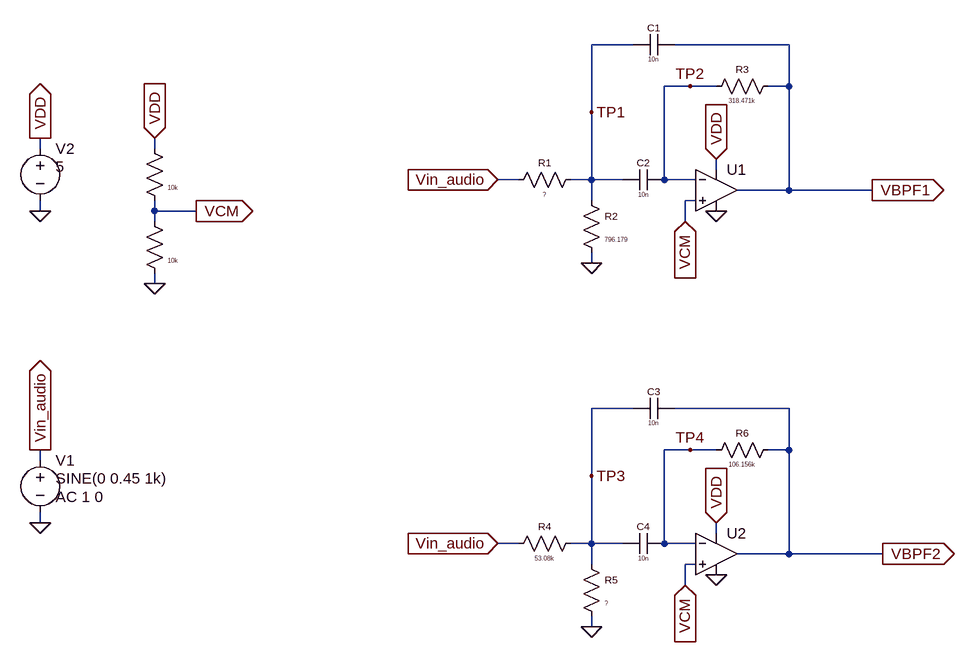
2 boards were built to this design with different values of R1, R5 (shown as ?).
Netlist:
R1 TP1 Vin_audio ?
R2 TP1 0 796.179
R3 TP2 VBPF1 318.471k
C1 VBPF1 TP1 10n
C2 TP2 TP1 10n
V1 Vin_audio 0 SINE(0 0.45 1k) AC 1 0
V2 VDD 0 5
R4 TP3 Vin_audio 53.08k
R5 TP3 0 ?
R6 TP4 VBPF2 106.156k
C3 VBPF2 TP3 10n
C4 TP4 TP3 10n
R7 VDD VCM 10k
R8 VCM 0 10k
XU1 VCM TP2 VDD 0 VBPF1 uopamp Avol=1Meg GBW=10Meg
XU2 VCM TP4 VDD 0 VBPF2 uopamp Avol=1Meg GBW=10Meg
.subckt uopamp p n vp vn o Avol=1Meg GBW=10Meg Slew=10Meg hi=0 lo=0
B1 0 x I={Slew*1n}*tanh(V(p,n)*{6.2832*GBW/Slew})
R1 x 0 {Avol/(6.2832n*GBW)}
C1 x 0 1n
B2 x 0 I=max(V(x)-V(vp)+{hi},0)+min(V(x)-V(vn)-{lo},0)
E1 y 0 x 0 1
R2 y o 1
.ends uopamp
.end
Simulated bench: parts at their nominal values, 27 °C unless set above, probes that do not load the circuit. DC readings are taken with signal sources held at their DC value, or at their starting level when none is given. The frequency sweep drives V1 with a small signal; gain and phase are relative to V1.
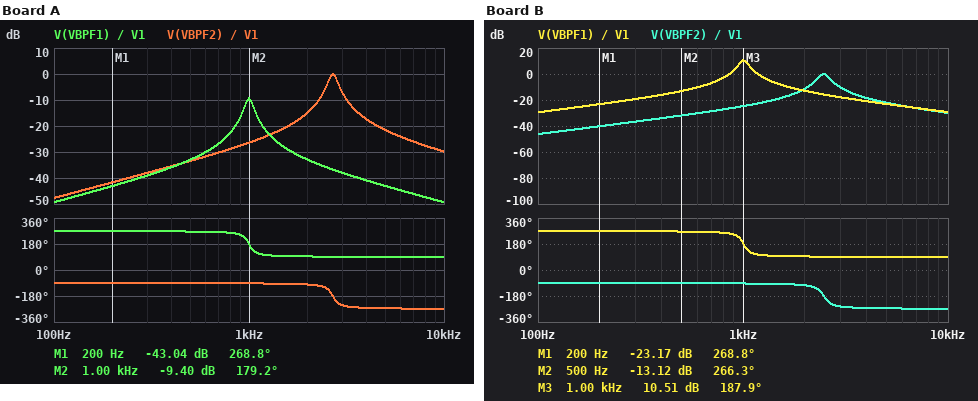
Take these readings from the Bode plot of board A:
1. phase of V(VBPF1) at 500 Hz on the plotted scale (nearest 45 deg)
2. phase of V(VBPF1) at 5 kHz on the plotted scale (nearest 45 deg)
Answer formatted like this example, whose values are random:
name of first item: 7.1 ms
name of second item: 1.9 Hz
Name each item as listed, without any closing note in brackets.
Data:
phase of V(VBPF1) at 500 Hz on the plotted scale: 270 deg
phase of V(VBPF1) at 5 kHz on the plotted scale: 90 deg
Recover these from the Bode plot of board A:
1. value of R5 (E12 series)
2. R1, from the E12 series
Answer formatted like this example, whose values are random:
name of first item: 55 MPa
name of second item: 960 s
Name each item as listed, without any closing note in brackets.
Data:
value of R5: 330 Ω
R1, from the E12 series: 470 kΩ
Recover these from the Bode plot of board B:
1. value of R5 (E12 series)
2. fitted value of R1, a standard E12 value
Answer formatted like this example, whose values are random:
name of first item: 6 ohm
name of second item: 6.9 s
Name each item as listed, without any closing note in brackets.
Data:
value of R5: 390 Ω
fitted value of R1, a standard E12 value: 47 kΩ
